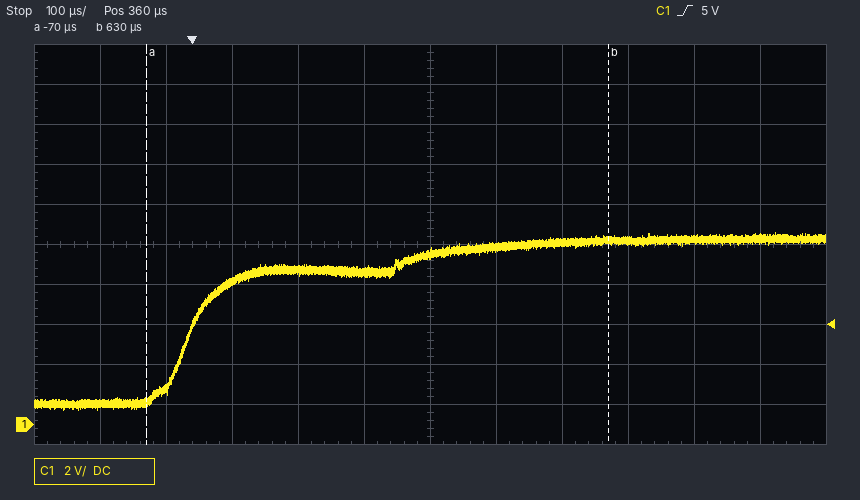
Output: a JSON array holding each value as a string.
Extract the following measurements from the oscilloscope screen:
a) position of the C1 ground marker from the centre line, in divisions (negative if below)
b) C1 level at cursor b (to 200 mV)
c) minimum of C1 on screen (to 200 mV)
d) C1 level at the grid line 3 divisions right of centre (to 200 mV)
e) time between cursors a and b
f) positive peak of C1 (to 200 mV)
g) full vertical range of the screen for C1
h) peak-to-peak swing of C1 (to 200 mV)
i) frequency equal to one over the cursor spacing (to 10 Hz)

["-4.5 div", "9.2 V", "800 mV", "9.2 V", "700 µs", "9.6 V", "20 V", "8.8 V", "1.43 kHz"]
